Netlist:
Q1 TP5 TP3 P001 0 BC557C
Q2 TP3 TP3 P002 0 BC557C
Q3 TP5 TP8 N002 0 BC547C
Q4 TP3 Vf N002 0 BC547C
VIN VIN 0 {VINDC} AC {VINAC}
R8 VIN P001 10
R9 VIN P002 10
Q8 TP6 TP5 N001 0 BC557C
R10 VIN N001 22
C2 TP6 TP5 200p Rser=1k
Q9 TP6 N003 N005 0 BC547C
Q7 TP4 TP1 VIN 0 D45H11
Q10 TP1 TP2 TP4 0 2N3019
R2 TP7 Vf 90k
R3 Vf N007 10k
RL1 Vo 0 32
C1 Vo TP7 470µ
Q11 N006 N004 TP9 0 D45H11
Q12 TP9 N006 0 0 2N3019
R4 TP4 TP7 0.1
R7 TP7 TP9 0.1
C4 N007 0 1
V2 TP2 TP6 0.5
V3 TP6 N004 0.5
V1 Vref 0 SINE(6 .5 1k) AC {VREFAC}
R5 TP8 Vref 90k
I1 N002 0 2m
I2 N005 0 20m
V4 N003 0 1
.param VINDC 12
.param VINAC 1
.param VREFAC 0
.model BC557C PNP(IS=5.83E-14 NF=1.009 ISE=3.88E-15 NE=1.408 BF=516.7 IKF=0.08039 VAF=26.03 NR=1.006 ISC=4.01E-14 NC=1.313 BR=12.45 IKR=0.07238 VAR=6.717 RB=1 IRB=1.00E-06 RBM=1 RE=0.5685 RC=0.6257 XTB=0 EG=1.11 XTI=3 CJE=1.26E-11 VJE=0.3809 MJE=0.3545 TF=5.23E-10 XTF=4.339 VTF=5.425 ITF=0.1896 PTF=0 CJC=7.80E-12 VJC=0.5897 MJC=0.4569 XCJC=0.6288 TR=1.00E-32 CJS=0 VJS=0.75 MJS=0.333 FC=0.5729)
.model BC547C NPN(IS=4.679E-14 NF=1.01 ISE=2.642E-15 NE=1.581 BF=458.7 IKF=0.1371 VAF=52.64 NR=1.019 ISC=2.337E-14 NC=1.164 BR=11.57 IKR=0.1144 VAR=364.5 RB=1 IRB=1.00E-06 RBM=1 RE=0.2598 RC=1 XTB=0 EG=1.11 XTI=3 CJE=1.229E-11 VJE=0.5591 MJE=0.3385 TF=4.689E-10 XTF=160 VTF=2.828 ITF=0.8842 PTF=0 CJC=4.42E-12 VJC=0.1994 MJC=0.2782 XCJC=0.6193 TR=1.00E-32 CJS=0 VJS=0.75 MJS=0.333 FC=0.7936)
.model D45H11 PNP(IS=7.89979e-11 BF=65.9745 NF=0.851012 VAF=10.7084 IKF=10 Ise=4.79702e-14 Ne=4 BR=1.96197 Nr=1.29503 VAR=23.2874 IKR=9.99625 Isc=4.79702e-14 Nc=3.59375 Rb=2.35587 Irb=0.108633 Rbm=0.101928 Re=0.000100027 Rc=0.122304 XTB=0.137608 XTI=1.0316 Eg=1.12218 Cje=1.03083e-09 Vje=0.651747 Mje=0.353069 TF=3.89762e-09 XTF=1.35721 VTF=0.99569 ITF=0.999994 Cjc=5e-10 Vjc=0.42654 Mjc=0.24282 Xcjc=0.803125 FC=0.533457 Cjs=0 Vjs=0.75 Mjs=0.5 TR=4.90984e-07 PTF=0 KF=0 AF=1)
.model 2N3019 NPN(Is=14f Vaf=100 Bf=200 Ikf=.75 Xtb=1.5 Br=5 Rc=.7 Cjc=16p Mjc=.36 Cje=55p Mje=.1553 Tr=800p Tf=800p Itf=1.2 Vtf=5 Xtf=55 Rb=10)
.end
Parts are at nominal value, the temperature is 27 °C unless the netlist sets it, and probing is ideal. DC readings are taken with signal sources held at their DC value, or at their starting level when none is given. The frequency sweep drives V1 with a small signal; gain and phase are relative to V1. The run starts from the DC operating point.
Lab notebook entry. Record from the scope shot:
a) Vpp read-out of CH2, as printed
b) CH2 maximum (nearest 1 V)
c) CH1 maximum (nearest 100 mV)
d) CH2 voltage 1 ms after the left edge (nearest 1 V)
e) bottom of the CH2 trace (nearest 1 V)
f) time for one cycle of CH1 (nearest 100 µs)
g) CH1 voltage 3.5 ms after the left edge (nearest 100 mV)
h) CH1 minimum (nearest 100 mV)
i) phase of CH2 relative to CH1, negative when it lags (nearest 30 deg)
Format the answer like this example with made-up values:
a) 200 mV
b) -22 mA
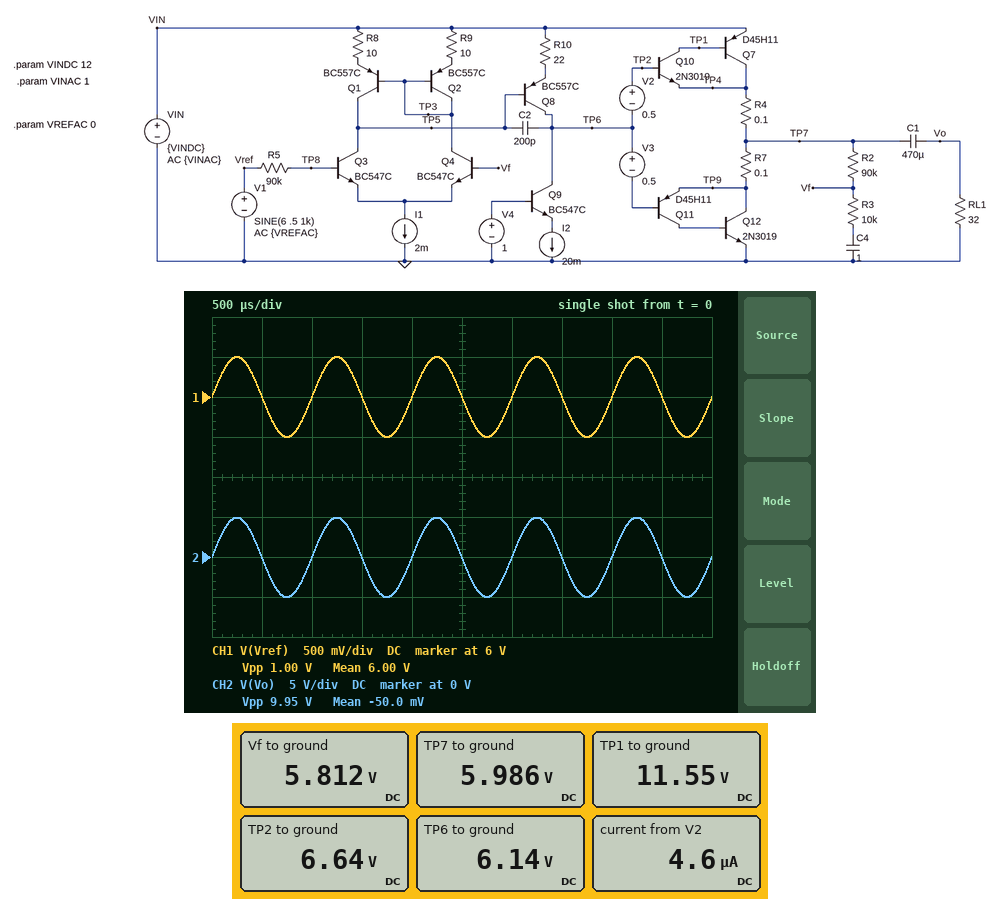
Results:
a) 9.95 V
b) 5 V
c) 6.5 V
d) 0 V
e) -5 V
f) 1.0 ms
g) 6.0 V
h) 5.5 V
i) 0 deg
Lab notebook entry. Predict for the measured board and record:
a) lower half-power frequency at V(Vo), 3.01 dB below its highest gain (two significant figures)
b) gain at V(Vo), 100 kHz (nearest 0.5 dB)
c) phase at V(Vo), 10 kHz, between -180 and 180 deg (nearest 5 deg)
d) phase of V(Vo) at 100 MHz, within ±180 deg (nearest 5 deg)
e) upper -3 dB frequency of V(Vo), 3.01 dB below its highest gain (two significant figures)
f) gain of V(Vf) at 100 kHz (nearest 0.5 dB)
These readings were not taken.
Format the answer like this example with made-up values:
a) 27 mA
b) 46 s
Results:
a) 11 Hz
b) 20.0 dB
c) 0 deg
d) 35 deg
e) 480 kHz
f) 0 dB
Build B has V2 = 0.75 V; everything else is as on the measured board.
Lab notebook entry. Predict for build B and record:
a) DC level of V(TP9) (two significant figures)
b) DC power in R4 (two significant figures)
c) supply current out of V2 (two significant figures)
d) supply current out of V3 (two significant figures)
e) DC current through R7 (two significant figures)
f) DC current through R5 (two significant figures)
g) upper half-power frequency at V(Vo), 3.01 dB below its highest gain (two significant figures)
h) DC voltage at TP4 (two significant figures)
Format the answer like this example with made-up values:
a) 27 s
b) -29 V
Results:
a) 5.9 V
b) 59 mW
c) 40 µA
d) 77 µA
e) 770 mA
f) 2.1 µA
g) 470 kHz
h) 6.1 V
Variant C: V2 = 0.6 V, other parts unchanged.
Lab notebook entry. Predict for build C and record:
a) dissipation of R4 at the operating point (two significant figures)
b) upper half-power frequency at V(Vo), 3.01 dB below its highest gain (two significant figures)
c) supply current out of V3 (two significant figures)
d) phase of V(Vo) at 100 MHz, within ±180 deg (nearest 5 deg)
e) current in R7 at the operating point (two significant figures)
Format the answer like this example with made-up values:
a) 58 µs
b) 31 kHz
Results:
a) 8.8 mW
b) 470 kHz
c) 20 µA
d) 20 deg
e) 300 mA
